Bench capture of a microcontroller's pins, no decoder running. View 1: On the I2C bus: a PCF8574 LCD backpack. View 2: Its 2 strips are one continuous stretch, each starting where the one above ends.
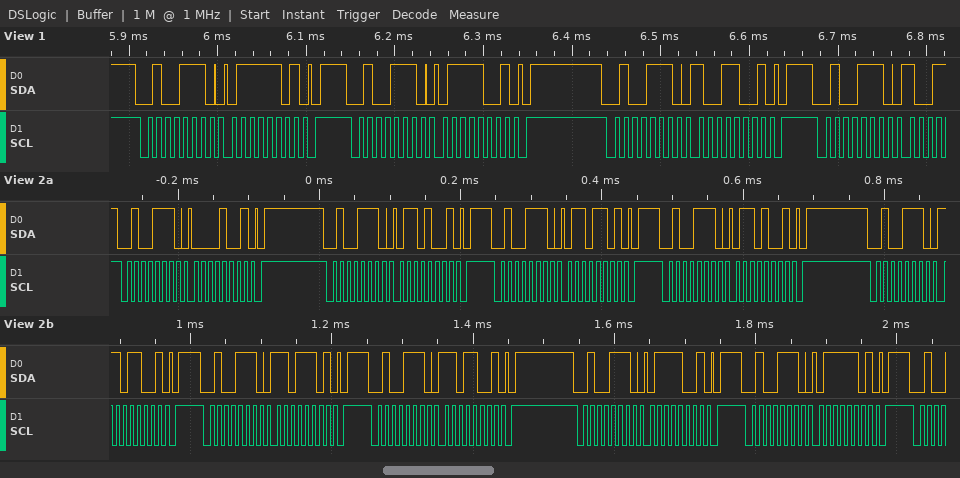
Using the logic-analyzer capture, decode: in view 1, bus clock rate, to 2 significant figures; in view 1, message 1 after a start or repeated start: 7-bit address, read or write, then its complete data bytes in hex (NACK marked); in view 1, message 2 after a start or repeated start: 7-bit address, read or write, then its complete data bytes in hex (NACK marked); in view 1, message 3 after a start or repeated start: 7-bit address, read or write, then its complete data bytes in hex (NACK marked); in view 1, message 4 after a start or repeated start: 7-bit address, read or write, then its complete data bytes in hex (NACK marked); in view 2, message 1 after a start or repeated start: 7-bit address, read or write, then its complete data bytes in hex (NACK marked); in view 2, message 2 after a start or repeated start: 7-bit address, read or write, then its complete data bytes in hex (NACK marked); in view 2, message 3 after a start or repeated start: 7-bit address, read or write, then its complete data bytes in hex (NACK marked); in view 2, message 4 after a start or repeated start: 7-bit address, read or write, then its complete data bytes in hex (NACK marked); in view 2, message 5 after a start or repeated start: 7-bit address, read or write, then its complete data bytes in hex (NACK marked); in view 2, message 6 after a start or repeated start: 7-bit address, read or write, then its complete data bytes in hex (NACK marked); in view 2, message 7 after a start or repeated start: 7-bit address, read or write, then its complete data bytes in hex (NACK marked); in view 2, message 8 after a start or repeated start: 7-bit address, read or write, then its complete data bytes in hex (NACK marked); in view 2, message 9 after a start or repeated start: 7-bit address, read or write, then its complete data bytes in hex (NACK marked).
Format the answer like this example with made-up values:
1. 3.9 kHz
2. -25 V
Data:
1. 100 kHz
2. 0x27 write: 7D
3. 0x27 write: 79
4. 0x27 write: 99
5. 0x27 write
6. 0x27 write: 09
7. 0x27 write: 69
8. 0x27 write: 6D
9. 0x27 write: 69
10. 0x27 write: D9
11. 0x27 write: DD
12. 0x27 write: D9
13. 0x27 write: 79
14. 0x27 write: 7D
